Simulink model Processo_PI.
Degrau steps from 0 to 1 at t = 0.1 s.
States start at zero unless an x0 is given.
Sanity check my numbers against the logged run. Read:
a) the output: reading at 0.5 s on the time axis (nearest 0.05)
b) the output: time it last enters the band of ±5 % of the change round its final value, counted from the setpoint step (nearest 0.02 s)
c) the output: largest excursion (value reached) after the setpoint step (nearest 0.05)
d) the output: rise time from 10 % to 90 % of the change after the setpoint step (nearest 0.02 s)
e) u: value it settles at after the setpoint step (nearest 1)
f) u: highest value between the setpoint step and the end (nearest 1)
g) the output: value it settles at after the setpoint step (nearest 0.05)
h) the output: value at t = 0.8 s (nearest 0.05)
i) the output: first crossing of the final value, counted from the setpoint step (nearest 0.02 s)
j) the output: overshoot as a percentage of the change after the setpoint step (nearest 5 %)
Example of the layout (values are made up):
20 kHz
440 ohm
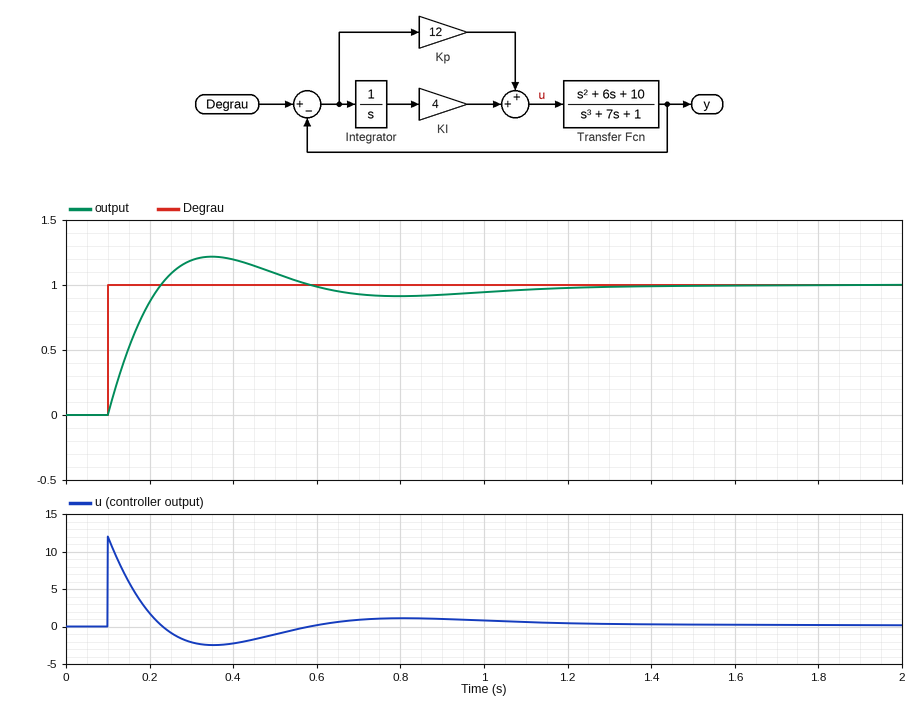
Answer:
1.10
0.92 s
1.20
0.10 s
0
12
1.00
0.90
0.12 s
20 %
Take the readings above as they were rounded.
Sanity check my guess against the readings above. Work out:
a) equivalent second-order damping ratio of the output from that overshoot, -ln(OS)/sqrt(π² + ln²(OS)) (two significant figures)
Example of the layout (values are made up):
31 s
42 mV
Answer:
0.46
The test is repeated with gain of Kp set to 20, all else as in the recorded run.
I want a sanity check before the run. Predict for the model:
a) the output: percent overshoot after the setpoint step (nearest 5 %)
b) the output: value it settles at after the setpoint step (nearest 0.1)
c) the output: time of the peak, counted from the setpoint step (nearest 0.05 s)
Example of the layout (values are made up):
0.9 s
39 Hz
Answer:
15 %
1.0
0.20 s
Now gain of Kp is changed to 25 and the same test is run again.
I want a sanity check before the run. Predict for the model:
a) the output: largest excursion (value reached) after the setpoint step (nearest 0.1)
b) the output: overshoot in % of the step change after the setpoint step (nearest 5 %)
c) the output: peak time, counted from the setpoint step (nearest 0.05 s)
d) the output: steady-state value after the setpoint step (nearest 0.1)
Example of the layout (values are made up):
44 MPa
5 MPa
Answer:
1.1
15 %
0.15 s
1.0
